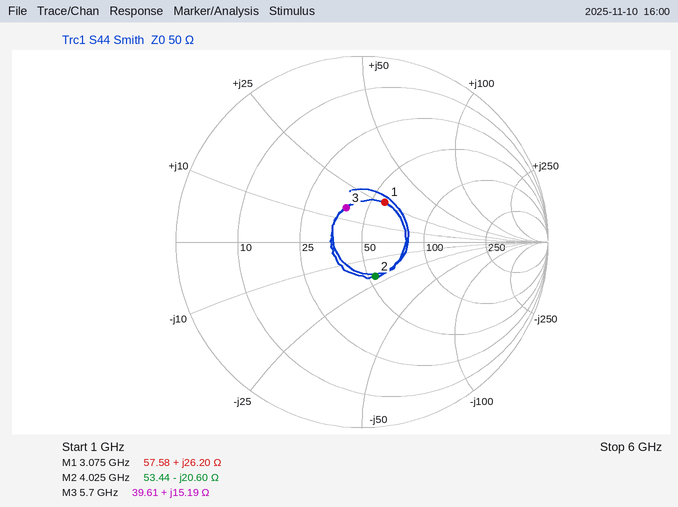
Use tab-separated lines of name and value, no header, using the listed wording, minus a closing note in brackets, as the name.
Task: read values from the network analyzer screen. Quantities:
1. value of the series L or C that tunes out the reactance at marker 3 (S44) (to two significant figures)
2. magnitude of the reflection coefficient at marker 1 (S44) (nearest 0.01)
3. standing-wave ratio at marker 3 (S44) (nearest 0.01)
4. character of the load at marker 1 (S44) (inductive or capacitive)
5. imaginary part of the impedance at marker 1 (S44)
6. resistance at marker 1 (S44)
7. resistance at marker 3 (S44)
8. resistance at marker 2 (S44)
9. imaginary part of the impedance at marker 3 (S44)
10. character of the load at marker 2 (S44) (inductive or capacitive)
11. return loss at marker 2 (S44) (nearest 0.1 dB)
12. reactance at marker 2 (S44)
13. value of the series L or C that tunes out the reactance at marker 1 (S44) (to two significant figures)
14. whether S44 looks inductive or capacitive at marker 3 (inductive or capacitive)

value of the series L or C that tunes out the reactance at marker 3 (S44)	1.8 pF
magnitude of the reflection coefficient at marker 1 (S44)	0.25
standing-wave ratio at marker 3 (S44)	1.51
character of the load at marker 1 (S44)	inductive
imaginary part of the impedance at marker 1	+26.20 Ω
resistance at marker 1	57.58 Ω
resistance at marker 3	39.61 Ω
resistance at marker 2	53.44 Ω
imaginary part of the impedance at marker 3	+15.19 Ω
character of the load at marker 2 (S44)	capacitive
return loss at marker 2 (S44)	14.1 dB
reactance at marker 2	-20.60 Ω
value of the series L or C that tunes out the reactance at marker 1 (S44)	2.0 pF
whether S44 looks inductive or capacitive at marker 3	inductive
